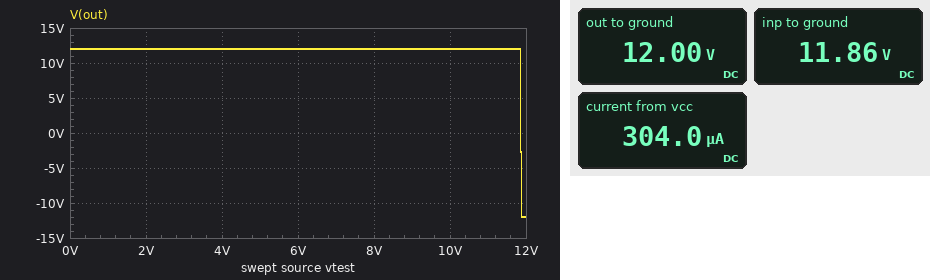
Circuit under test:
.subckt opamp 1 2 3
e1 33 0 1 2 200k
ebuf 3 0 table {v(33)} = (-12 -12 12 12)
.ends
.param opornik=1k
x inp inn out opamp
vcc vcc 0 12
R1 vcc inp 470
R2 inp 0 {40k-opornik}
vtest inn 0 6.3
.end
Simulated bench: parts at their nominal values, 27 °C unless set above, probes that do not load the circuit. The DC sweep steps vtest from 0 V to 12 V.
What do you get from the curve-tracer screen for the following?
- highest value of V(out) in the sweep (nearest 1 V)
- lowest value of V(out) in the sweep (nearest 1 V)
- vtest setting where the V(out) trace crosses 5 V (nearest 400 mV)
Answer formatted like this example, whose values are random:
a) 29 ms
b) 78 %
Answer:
a) 12 V
b) -12 V
c) 12.0 V
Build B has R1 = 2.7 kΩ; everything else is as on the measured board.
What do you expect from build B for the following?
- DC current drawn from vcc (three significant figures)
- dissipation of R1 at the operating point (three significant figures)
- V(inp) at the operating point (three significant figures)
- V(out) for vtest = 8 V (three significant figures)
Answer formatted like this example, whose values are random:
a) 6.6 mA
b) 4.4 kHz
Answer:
a) 288 µA
b) 224 µW
c) 11.2 V
d) 12.0 V
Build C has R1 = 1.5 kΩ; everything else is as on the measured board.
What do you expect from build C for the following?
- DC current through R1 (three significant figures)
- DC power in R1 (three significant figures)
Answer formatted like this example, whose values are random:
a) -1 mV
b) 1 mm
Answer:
a) 296 µA
b) 132 µW
